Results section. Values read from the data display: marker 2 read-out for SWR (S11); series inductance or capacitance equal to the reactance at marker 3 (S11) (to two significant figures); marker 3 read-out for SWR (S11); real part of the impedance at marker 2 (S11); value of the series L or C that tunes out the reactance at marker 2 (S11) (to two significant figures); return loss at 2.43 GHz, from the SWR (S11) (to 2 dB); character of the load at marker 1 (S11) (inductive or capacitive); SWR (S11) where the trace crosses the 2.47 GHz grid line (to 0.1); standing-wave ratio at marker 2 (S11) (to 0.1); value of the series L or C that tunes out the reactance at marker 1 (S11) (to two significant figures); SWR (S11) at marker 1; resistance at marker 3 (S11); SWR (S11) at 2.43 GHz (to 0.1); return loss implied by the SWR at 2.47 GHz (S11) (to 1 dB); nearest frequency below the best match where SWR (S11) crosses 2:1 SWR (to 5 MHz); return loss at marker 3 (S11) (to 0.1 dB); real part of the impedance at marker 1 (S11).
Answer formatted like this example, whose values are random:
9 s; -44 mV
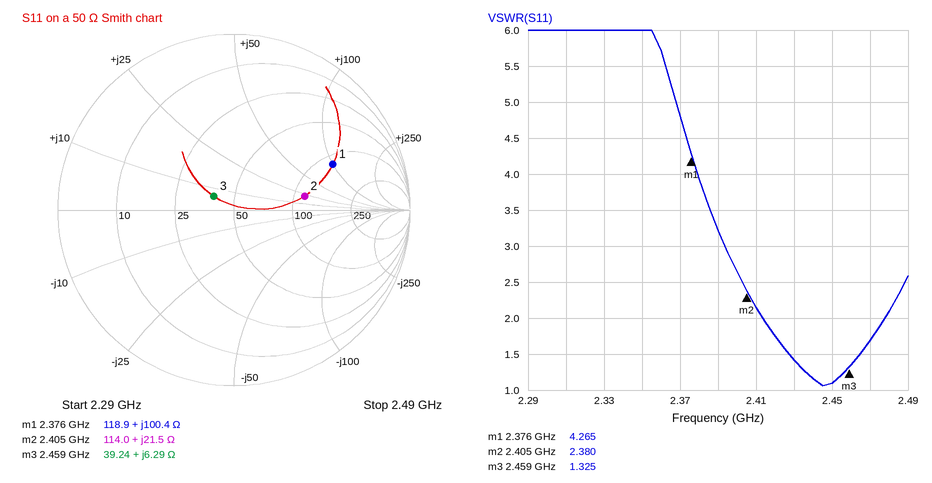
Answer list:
2.380; 410 pH; 1.325; 114.0 Ω; 3.1 pF; 16 dB; inductive; 1.7; 2.4; 670 fF; 4.265; 39.24 Ω; 1.4; 12 dB; 2.415 GHz; 17.1 dB; 118.9 Ω
